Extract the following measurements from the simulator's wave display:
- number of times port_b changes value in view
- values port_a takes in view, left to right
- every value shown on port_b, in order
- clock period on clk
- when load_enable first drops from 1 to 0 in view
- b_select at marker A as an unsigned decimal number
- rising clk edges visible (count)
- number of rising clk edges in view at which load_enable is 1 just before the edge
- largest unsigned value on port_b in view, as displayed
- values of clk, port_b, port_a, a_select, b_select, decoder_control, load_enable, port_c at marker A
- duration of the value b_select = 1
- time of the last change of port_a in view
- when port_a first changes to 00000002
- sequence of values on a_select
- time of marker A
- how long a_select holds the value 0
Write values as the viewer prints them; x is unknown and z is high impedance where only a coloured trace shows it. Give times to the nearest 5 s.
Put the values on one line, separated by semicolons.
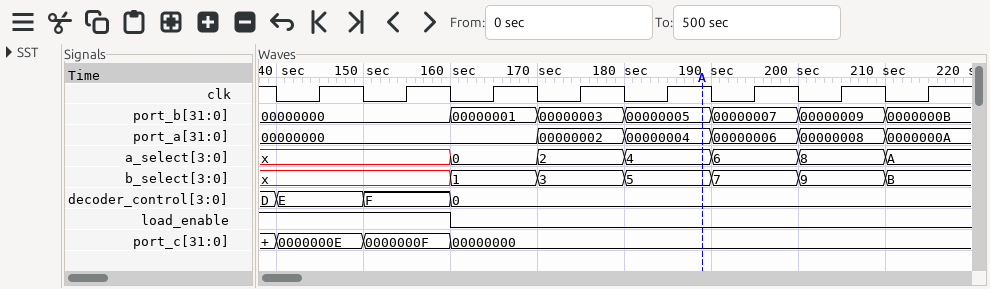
6; 00000000, 00000002, 00000004, 00000006, 00000008, 0000000A; 00000000, 00000001, 00000003, 00000005, 00000007, 00000009, 0000000B; 10 s; 160 s; 5; 8; 2; 0000000B; clk=1, port_b=00000005, port_a=00000004, a_select=4, b_select=5, decoder_control=0, load_enable=0, port_c=00000000; 10 s; 210 s; 170 s; x, 0, 2, 4, 6, 8, A; 190 s; 10 s
